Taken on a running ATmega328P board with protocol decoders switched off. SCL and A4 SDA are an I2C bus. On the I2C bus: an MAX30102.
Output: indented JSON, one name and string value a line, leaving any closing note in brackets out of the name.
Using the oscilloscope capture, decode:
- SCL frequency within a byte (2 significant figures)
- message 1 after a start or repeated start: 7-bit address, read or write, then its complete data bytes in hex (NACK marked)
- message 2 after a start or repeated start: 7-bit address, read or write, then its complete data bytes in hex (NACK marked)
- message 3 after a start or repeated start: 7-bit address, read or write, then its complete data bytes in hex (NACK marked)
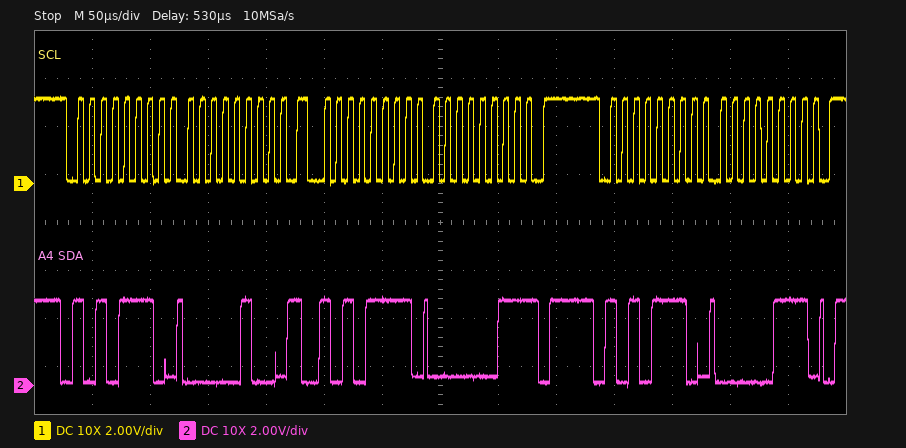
{
  "SCL frequency within a byte": "100 kHz",
  "message 1 after a start or repeated start: 7-bit address, read or write, then its complete data bytes in hex": "0x57 write: 04",
  "message 2 after a start or repeated start: 7-bit address, read or write, then its complete data bytes in hex": "0x57 read: 03 NACK",
  "message 3 after a start or repeated start: 7-bit address, read or write, then its complete data bytes in hex": "0x57 write: 07"
}
